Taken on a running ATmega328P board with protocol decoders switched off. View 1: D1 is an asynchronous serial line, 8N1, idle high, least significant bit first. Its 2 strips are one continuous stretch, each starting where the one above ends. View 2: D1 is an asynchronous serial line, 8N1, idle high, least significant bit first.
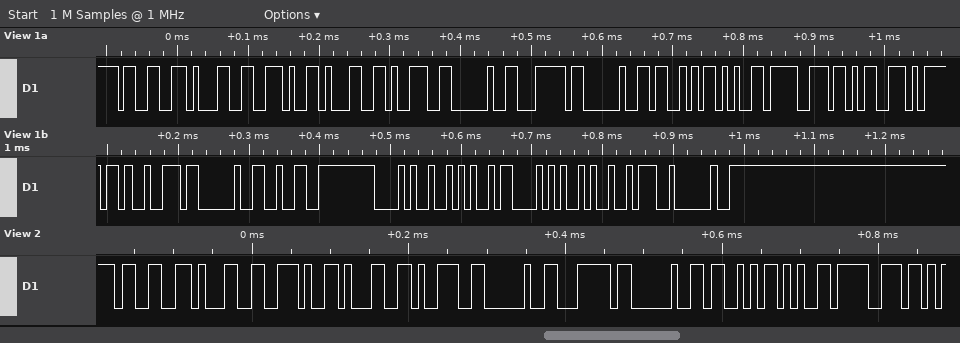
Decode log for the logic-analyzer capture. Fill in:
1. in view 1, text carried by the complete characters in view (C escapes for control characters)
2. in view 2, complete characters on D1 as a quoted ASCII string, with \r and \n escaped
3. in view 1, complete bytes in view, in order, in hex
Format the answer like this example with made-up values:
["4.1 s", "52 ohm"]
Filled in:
["\"31.19 | Sensor 2(*C): \"", "\"31.19 | Sen\"", "0x33 0x31 0x2E 0x31 0x39 0x20 0x7C 0x20 0x53 0x65 0x6E 0x73 0x6F 0x72 0x20 0x32 0x28 0x2A 0x43 0x29 0x3A 0x20"]
